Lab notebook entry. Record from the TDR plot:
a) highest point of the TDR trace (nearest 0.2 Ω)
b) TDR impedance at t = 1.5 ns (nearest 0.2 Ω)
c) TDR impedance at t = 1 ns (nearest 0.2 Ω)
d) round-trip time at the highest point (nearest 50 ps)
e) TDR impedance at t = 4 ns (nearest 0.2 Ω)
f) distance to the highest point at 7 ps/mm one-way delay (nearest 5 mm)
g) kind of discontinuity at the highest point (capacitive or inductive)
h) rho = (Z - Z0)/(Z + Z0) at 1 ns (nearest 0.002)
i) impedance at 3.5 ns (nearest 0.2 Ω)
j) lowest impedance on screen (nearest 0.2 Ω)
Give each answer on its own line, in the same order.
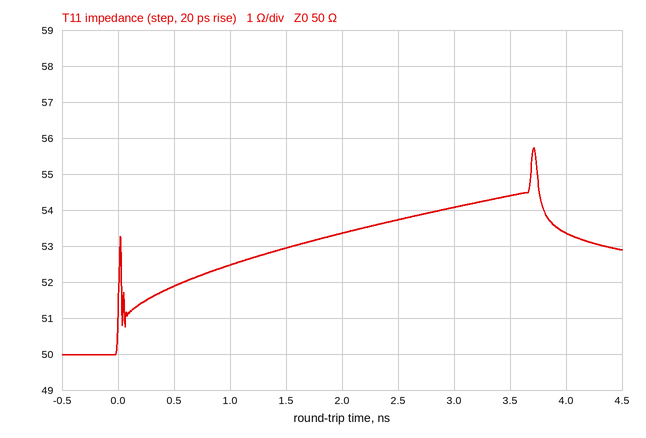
55.8 Ω
53.0 Ω
52.4 Ω
3.70 ns
53.4 Ω
265 mm
inductive
+0.024
54.4 Ω
50.0 Ω
